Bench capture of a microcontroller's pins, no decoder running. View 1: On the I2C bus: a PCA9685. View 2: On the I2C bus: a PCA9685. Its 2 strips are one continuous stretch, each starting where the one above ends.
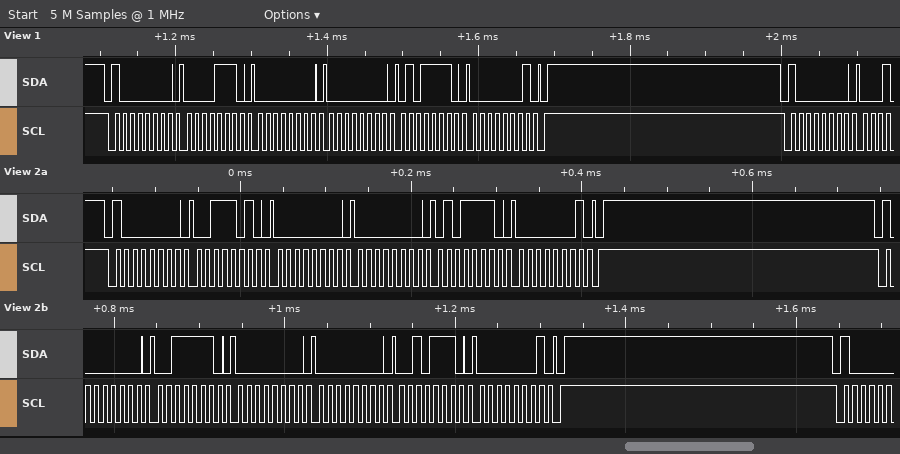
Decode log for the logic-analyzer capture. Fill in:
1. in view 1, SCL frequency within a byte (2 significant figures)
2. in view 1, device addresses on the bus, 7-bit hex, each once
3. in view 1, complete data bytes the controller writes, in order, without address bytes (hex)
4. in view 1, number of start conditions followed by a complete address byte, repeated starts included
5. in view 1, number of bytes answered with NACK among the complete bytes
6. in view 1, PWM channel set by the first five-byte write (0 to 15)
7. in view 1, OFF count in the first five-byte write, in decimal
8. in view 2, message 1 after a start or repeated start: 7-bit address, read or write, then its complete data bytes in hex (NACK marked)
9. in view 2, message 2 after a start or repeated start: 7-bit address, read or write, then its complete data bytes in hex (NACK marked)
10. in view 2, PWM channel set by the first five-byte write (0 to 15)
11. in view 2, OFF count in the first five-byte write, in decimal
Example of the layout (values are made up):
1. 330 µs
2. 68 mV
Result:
1. 100 kHz
2. 0x40
3. 0E 00 00 5E 01
4. 2
5. 0
6. 2
7. 350
8. 0x40 write: 3A 00 00 5E 01
9. 0x40 write: 3E 00 00 2E 01
10. 13
11. 350
